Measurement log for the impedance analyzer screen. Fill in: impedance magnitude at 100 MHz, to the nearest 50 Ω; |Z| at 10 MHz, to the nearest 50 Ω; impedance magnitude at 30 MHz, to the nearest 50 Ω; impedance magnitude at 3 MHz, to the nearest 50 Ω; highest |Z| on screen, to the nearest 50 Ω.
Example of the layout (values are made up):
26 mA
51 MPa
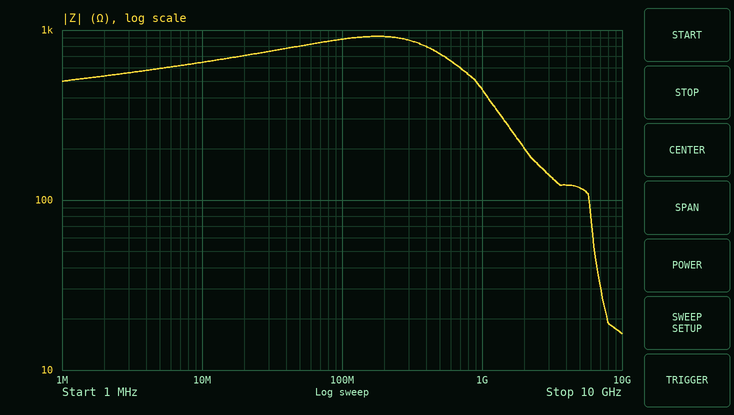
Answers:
900 Ω
650 Ω
750 Ω
550 Ω
900 Ω
